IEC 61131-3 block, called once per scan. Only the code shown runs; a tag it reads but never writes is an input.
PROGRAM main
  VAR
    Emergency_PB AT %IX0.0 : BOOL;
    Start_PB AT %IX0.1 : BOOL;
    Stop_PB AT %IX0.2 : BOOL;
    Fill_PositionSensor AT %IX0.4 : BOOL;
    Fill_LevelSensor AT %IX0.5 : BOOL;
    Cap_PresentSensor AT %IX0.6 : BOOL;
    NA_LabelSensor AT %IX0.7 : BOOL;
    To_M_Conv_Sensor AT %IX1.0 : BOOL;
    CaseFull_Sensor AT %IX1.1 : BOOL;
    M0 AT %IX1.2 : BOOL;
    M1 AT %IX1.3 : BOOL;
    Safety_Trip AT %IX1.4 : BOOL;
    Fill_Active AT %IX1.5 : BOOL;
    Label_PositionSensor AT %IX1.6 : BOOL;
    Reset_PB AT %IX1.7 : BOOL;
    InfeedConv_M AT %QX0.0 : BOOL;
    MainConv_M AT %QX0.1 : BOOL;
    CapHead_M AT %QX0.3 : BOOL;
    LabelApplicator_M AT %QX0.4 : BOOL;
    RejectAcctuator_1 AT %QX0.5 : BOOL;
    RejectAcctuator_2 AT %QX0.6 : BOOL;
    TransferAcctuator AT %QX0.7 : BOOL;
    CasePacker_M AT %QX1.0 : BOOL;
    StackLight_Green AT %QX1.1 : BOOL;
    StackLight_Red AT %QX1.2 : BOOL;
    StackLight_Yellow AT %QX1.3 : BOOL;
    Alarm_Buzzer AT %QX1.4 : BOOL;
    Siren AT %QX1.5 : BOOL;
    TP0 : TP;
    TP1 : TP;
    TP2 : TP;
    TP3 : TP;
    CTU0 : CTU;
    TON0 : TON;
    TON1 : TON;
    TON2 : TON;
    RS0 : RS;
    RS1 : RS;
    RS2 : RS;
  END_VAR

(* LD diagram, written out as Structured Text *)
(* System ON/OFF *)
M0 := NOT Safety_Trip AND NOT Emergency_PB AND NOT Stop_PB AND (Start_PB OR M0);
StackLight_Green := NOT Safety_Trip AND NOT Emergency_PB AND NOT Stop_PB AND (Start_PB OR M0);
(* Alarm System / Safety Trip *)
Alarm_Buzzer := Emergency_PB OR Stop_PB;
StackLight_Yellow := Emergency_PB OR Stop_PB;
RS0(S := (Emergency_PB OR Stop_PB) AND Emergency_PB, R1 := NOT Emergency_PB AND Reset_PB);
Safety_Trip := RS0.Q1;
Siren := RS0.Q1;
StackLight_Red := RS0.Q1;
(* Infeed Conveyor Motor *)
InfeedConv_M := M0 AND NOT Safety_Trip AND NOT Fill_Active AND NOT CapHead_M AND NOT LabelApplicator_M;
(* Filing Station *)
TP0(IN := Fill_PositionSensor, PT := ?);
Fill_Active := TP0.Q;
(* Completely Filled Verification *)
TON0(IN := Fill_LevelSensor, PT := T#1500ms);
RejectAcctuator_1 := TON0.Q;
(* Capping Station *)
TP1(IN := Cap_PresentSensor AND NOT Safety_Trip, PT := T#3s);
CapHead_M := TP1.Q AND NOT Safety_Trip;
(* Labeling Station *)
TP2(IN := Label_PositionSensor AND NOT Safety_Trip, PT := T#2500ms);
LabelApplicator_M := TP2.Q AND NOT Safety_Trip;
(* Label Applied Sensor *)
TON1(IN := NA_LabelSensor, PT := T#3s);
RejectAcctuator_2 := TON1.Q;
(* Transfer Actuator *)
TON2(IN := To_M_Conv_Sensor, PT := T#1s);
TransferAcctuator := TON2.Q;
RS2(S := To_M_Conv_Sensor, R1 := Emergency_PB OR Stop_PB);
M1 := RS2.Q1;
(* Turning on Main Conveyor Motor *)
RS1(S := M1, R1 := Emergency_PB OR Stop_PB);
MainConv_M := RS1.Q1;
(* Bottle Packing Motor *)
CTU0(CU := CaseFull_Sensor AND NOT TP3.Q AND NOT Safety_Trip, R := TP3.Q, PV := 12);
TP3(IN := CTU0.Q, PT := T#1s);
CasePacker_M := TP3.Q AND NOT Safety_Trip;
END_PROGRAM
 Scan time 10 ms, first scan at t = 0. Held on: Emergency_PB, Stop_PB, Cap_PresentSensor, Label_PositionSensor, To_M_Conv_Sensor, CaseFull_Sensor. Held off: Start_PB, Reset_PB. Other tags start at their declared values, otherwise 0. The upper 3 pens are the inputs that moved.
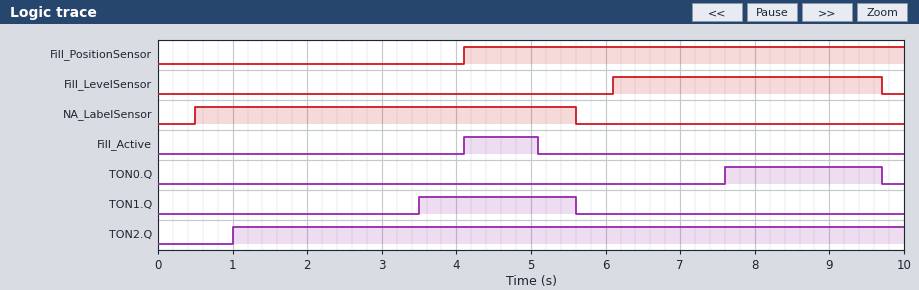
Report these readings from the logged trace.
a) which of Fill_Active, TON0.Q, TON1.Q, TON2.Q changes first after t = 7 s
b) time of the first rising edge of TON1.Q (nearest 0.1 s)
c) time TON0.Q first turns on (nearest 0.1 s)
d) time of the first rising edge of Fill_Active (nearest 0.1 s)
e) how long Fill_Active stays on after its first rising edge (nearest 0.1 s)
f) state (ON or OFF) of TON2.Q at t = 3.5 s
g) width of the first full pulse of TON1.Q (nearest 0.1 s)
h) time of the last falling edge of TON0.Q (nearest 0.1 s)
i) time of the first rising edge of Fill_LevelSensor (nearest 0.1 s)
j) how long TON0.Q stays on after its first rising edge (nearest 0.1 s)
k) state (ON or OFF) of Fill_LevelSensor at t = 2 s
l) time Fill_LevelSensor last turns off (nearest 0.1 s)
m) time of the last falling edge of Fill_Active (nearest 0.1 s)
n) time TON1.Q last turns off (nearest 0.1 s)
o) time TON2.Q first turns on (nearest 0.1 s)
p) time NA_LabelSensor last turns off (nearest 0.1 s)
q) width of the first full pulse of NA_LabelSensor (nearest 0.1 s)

TON0.Q
3.5 s
7.6 s
4.1 s
1.0 s
ON
2.1 s
9.7 s
6.1 s
2.1 s
OFF
9.7 s
5.1 s
5.6 s
1.0 s
5.6 s
5.1 s
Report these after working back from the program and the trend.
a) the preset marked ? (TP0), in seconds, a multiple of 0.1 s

1.0 s
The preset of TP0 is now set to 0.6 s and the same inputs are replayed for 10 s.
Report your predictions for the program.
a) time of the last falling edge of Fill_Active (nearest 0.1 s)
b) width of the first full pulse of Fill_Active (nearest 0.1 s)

4.7 s
0.6 s
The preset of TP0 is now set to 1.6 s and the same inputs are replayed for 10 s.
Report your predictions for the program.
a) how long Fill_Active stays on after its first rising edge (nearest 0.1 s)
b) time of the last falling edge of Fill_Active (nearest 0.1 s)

1.6 s
5.7 s
